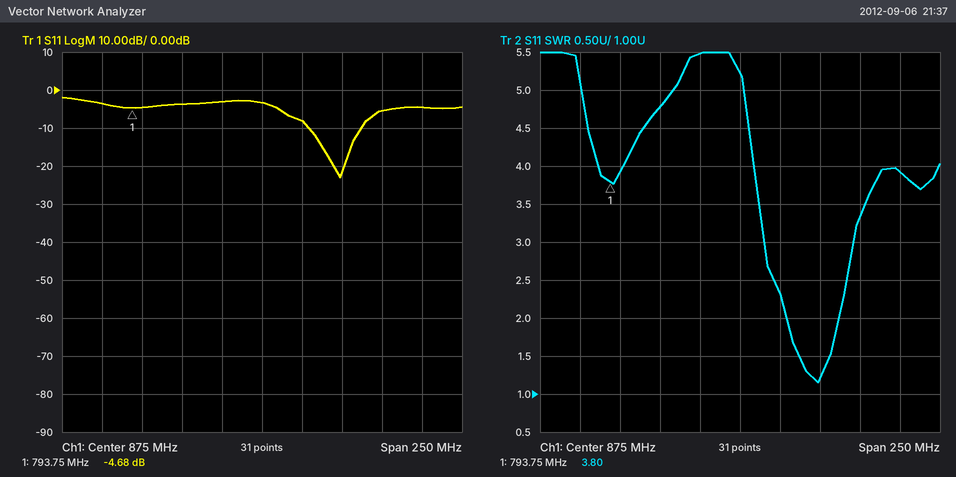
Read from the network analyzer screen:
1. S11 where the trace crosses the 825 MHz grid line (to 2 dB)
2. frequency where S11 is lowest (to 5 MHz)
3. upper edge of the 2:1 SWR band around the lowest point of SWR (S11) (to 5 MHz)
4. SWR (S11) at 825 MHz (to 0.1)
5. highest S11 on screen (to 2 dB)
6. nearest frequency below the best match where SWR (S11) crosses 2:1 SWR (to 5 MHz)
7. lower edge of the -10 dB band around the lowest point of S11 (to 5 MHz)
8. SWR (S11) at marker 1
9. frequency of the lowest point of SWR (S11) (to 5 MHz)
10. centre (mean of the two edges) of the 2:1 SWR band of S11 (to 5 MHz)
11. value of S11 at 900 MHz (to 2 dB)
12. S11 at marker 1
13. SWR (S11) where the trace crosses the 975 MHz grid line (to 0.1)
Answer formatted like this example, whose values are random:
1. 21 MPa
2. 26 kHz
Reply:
1. -4 dB
2. 925 MHz
3. 935 MHz
4. 4.8
5. -2 dB
6. 905 MHz
7. 905 MHz
8. 3.80
9. 925 MHz
10. 920 MHz
11. -8 dB
12. -4.68 dB
13. 3.9
